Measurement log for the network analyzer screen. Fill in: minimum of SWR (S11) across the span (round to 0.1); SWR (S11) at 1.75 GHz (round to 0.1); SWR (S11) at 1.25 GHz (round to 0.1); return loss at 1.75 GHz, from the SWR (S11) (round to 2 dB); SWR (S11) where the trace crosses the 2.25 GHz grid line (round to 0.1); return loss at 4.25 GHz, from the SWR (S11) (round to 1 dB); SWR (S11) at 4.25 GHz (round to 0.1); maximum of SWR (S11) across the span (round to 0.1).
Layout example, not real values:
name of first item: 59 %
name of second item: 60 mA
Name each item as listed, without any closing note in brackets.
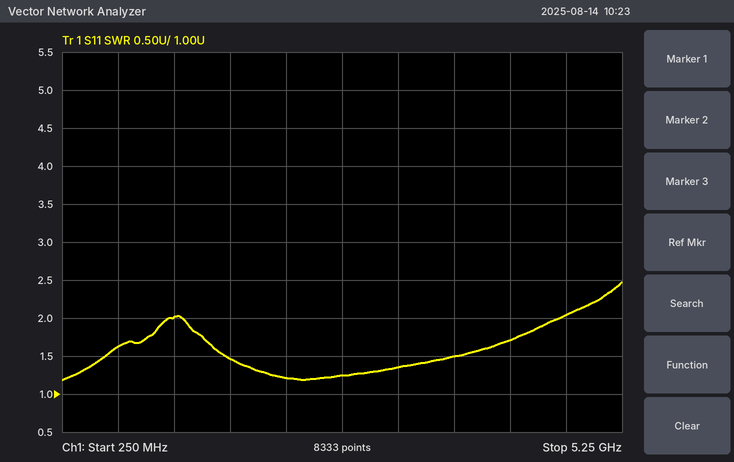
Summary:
minimum of SWR (S11) across the span: 1.2
SWR (S11) at 1.75 GHz: 1.5
SWR (S11) at 1.25 GHz: 2.0
return loss at 1.75 GHz, from the SWR (S11): 14 dB
SWR (S11) where the trace crosses the 2.25 GHz grid line: 1.2
return loss at 4.25 GHz, from the SWR (S11): 12 dB
SWR (S11) at 4.25 GHz: 1.7
maximum of SWR (S11) across the span: 2.5
